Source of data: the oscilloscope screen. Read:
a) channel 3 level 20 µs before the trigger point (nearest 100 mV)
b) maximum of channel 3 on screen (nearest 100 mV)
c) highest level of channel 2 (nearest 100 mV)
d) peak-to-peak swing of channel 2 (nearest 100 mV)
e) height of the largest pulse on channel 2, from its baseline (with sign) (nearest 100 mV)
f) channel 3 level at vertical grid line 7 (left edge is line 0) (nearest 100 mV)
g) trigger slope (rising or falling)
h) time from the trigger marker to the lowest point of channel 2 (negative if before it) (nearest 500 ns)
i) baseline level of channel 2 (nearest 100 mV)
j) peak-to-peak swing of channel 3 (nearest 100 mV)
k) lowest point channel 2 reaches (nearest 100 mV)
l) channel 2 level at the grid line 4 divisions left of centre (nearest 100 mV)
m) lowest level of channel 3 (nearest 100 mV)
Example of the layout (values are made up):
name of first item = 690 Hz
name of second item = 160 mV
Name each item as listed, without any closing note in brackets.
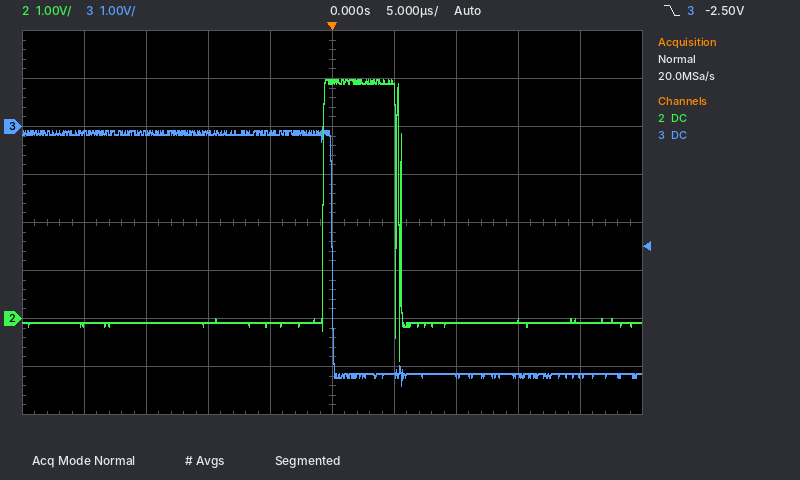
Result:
channel 3 level 20 µs before the trigger point = -100 mV
maximum of channel 3 on screen = 0.0 V
highest level of channel 2 = 5.0 V
peak-to-peak swing of channel 2 = 5.9 V
height of the largest pulse on channel 2, from its baseline (with sign) = +5.1 V
channel 3 level at vertical grid line 7 (left edge is line 0) = -5.2 V
trigger slope = falling
time from the trigger marker to the lowest point of channel 2 (negative if before it) = +5.5 µs
baseline level of channel 2 = -100 mV
peak-to-peak swing of channel 3 = 5.4 V
lowest point channel 2 reaches = -900 mV
channel 2 level at the grid line 4 divisions left of centre = -100 mV
lowest level of channel 3 = -5.4 V
